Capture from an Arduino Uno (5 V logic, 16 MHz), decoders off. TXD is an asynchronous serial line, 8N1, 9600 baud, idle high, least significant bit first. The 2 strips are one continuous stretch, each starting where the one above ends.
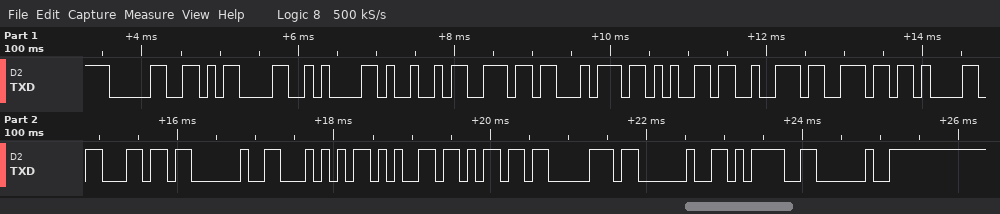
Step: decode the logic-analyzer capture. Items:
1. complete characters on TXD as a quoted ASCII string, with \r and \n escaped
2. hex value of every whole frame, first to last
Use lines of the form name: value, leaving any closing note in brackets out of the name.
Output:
complete characters on TXD as a quoted ASCII string, with \r and \n escaped: "0\r\nInternal Temp = "
hex value of every whole frame, first to last: 0x30 0x0D 0x0A 0x49 0x6E 0x74 0x65 0x72 0x6E 0x61 0x6C 0x20 0x54 0x65 0x6D 0x70 0x20 0x3D 0x20
